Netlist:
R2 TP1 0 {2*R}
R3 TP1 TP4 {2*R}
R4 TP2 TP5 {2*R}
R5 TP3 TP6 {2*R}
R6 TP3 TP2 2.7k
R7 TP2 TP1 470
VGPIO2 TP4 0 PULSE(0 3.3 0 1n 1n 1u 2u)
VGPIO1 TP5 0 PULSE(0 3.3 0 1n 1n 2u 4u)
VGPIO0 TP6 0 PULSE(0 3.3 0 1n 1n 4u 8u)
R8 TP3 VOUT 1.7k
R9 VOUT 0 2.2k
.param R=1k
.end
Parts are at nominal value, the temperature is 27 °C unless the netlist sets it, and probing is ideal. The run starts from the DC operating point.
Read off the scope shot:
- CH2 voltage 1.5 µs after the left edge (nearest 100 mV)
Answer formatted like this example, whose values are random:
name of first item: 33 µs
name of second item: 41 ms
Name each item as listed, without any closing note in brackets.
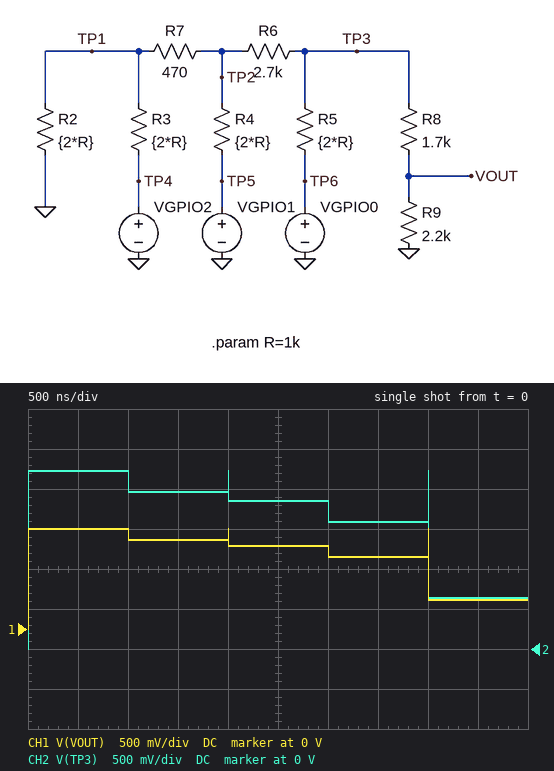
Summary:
CH2 voltage 1.5 µs after the left edge: 2.0 V
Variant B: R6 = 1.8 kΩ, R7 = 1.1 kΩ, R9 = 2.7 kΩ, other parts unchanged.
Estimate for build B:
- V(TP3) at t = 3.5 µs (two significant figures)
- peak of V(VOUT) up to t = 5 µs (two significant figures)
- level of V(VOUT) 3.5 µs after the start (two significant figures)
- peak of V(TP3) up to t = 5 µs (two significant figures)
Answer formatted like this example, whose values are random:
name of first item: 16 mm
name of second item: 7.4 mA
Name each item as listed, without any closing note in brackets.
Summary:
V(TP3) at t = 3.5 µs: 1.5 V
peak of V(VOUT) up to t = 5 µs: 1.4 V
level of V(VOUT) 3.5 µs after the start: 940 mV
peak of V(TP3) up to t = 5 µs: 2.3 V
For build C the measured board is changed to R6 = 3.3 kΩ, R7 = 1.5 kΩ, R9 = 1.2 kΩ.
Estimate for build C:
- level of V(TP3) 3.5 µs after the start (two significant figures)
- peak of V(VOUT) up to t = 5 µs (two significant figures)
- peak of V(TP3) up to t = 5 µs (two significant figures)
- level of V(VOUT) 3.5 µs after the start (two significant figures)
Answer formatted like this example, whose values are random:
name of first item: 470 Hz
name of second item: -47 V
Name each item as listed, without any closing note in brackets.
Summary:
level of V(TP3) 3.5 µs after the start: 1.5 V
peak of V(VOUT) up to t = 5 µs: 860 mV
peak of V(TP3) up to t = 5 µs: 2.1 V
level of V(VOUT) 3.5 µs after the start: 640 mV
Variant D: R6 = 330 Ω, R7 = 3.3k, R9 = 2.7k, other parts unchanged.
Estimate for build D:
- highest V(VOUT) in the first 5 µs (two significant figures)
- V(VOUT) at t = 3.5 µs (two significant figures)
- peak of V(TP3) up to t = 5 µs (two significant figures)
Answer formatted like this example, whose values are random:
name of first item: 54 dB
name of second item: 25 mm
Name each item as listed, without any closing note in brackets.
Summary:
highest V(VOUT) in the first 5 µs: 1.5 V
V(VOUT) at t = 3.5 µs: 770 mV
peak of V(TP3) up to t = 5 µs: 2.5 V
